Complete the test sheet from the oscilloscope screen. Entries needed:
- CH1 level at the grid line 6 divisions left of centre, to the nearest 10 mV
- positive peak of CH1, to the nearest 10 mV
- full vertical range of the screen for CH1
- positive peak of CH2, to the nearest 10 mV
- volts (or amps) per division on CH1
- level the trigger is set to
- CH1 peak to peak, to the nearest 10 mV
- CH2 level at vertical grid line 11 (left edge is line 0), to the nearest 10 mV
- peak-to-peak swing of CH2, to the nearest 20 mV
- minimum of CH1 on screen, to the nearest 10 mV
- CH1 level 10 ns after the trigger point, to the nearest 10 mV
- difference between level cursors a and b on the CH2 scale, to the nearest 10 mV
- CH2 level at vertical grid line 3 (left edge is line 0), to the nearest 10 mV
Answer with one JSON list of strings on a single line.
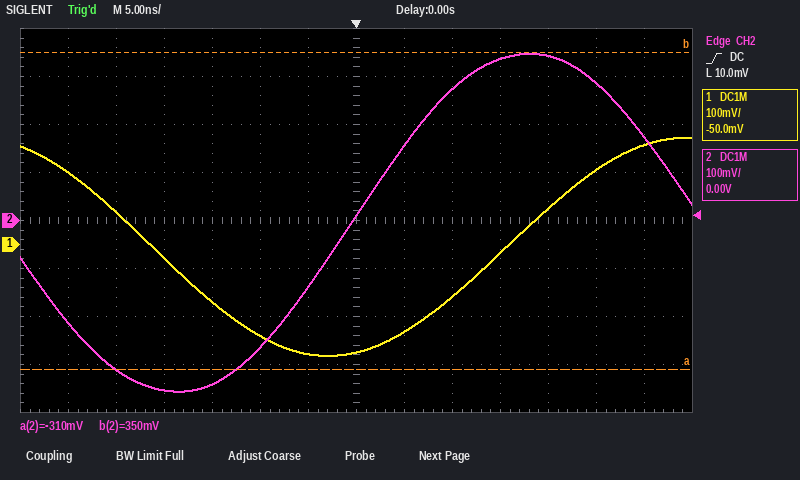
["150 mV", "220 mV", "800 mV", "350 mV", "100 mV", "10.0 mV", "450 mV", "340 mV", "700 mV", "-230 mV", "-110 mV", "660 mV", "-350 mV"]
